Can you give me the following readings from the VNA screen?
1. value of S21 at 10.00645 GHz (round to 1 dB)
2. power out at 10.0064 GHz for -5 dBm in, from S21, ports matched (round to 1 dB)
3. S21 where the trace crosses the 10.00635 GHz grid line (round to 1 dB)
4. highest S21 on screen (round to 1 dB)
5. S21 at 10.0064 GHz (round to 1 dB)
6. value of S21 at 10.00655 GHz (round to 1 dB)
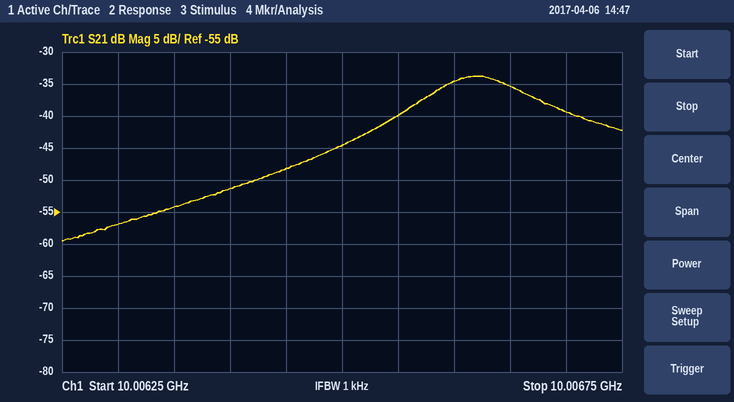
-48 dB
-56 dBm
-54 dB
-34 dB
-51 dB
-40 dB
